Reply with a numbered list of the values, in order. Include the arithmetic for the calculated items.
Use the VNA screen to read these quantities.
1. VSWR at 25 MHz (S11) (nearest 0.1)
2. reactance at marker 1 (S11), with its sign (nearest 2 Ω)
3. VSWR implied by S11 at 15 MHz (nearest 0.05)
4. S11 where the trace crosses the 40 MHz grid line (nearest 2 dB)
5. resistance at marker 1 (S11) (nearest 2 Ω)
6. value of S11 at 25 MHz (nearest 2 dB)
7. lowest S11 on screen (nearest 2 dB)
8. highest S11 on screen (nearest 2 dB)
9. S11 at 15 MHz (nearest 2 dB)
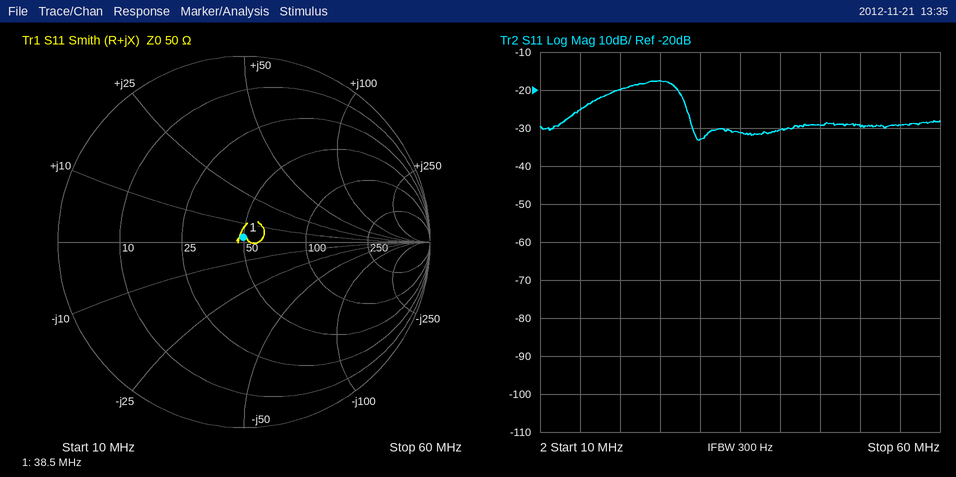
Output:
1. |Γ| = 10^(-18/20) = 0.1259; VSWR = (1 + 0.1259)/(1 − 0.1259) ≈ 1.3
2. +2 Ω
3. |Γ| = 10^(-26/20) = 0.0501; VSWR = (1 + 0.0501)/(1 − 0.0501) ≈ 1.11, so 1.10 to the nearest 0.05
4. -30 dB
5. 50 Ω
6. -18 dB
7. -34 dB
8. -18 dB
9. -26 dB
